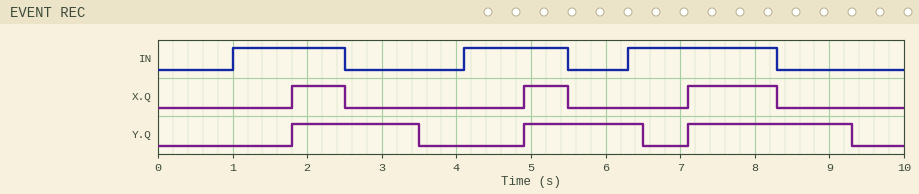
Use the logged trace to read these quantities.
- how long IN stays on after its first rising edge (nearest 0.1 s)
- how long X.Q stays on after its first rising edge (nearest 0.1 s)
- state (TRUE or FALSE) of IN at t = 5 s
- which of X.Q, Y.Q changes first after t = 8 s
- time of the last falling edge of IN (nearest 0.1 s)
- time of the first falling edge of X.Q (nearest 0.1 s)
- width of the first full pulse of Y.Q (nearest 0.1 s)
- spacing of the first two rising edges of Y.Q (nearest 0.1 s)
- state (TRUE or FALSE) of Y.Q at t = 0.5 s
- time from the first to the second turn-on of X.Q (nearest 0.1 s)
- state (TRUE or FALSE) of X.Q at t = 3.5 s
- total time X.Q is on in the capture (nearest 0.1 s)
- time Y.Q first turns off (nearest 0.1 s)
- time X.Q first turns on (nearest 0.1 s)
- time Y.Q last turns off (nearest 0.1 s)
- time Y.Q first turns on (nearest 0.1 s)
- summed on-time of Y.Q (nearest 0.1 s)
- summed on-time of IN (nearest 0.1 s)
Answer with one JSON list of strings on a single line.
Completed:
["1.5 s", "0.7 s", "TRUE", "X.Q", "8.3 s", "2.5 s", "1.7 s", "3.1 s", "FALSE", "3.1 s", "FALSE", "2.5 s", "3.5 s", "1.8 s", "9.3 s", "1.8 s", "5.5 s", "4.9 s"]
